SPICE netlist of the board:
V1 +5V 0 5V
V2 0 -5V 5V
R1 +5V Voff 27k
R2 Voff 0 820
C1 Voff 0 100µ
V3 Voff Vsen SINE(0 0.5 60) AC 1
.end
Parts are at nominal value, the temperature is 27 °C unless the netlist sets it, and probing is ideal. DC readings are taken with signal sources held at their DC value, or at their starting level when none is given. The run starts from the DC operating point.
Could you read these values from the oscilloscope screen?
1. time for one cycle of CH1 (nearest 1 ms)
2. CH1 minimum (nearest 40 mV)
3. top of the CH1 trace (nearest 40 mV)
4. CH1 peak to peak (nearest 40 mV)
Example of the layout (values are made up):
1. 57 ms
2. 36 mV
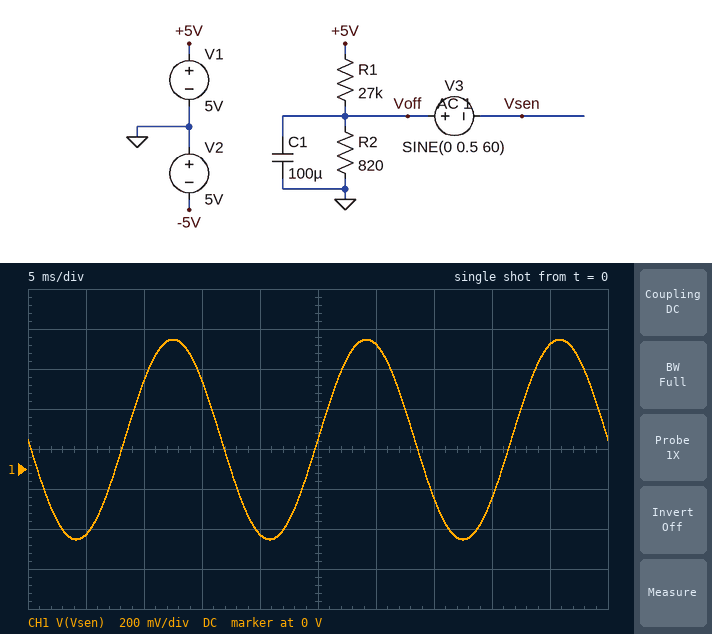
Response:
1. 17 ms
2. -360 mV
3. 640 mV
4. 1.00 V
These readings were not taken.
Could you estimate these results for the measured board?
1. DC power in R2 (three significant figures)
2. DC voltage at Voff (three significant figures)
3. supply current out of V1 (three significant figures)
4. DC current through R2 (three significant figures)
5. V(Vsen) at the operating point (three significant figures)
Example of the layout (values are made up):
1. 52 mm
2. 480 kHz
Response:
1. 26.5 µW
2. 147 mV
3. 180 µA
4. 180 µA
5. 147 mV
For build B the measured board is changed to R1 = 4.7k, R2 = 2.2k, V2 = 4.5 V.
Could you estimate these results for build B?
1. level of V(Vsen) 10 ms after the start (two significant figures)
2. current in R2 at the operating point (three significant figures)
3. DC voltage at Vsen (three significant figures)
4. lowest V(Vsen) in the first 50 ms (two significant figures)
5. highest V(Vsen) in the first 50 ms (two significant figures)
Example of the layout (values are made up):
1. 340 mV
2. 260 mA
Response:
1. 1.9 V
2. 725 µA
3. 1.59 V
4. 1.1 V
5. 2.1 V
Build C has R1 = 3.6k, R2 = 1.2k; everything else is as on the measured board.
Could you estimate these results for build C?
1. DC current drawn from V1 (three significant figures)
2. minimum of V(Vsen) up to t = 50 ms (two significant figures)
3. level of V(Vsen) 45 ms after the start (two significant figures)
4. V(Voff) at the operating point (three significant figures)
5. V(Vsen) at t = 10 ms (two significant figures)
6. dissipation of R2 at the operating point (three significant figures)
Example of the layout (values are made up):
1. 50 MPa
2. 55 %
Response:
1. 1.04 mA
2. 750 mV
3. 1.7 V
4. 1.25 V
5. 1.5 V
6. 1.30 mW
